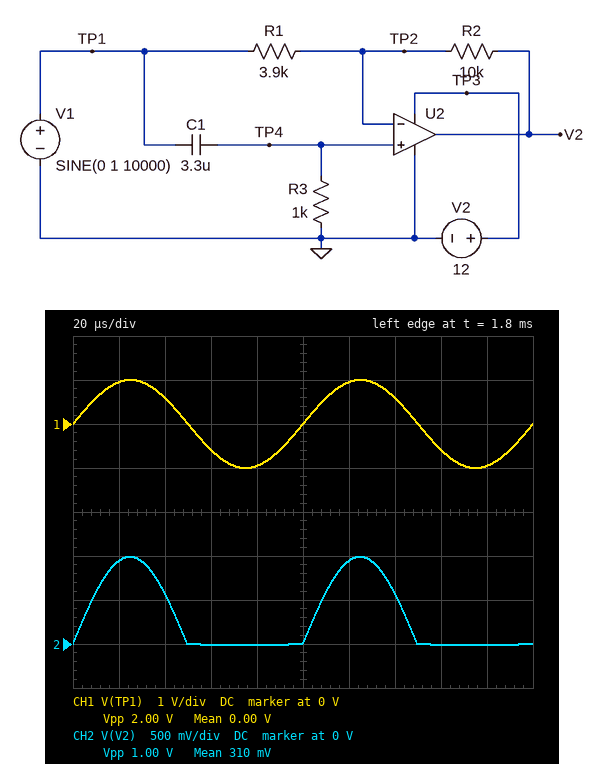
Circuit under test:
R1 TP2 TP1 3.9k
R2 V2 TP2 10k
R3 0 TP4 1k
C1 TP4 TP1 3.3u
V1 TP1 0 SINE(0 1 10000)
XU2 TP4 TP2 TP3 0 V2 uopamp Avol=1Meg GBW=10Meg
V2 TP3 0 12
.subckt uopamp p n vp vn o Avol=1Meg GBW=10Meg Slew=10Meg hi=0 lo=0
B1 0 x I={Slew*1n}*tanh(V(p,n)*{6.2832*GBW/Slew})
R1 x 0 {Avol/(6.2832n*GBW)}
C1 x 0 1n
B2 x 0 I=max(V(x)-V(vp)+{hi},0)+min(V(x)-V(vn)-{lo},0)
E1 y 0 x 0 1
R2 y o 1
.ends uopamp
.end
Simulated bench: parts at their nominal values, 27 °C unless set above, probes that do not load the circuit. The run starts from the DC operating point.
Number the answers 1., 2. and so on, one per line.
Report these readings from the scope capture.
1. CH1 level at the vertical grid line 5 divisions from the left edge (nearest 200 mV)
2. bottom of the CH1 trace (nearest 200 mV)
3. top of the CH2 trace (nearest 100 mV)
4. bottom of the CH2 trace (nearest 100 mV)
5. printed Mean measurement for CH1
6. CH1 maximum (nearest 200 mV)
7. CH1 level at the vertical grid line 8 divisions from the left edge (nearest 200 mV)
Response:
1. 0 V
2. -1.0 V
3. 1.0 V
4. 0 V
5. 0.00 V
6. 1.0 V
7. -600 mV
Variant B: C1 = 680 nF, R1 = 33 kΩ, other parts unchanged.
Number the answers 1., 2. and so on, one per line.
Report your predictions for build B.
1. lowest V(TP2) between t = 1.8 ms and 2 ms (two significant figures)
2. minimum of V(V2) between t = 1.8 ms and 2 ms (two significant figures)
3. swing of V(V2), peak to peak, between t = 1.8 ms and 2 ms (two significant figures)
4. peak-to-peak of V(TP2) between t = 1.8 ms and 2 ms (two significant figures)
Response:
1. -240 mV
2. -10 mV
3. 1.0 V
4. 1.2 V
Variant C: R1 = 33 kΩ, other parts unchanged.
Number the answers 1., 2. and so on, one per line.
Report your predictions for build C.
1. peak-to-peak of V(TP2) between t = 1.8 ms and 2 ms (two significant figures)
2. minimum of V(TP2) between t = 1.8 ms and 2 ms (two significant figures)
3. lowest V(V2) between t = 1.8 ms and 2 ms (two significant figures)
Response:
1. 1.2 V
2. -240 mV
3. -10 mV
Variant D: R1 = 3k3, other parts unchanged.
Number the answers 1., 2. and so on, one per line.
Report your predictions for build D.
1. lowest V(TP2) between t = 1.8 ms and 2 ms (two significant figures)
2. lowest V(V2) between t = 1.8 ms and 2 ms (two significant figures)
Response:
1. -750 mV
2. -9.2 mV
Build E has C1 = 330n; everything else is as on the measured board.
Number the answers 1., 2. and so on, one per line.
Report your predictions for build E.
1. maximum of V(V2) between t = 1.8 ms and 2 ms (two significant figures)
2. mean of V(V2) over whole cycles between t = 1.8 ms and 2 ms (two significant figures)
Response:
1. 1.0 V
2. 320 mV
